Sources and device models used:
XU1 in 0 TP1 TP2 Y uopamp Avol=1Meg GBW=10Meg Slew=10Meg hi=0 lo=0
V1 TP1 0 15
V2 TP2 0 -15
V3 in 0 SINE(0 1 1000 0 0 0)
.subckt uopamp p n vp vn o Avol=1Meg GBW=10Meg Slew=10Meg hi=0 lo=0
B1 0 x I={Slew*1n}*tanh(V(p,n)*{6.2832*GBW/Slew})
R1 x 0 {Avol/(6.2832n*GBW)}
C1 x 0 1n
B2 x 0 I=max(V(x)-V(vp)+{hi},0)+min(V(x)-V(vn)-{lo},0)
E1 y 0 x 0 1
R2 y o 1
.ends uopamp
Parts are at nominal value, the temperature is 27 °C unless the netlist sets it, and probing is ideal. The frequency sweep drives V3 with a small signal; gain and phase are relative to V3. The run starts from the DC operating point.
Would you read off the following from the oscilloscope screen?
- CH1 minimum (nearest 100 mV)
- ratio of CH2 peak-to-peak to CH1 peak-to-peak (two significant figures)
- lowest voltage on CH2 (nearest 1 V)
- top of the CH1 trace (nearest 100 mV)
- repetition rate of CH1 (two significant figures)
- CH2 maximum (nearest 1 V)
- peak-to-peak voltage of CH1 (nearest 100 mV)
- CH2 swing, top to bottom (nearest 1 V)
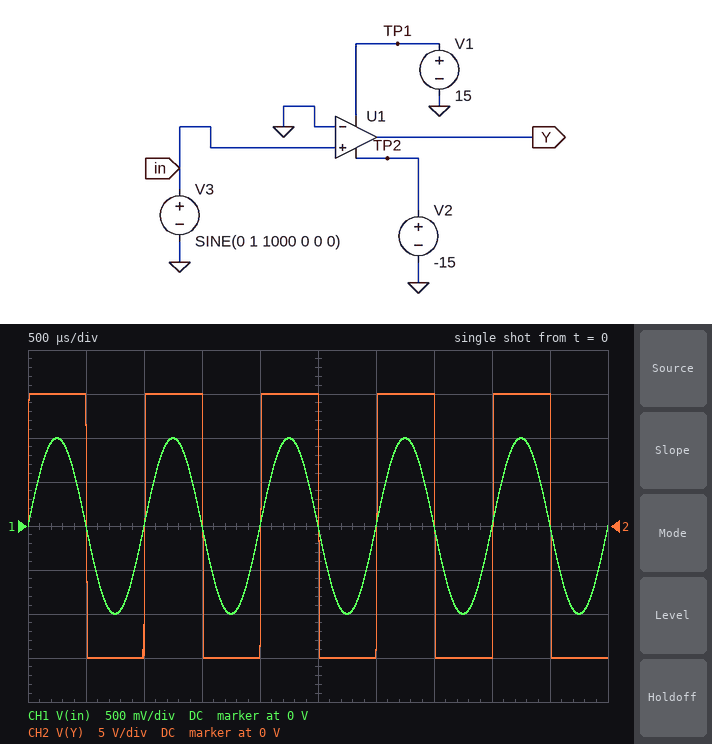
-1.0 V
15
-15 V
1.0 V
1.0 kHz
15 V
2.0 V
30 V
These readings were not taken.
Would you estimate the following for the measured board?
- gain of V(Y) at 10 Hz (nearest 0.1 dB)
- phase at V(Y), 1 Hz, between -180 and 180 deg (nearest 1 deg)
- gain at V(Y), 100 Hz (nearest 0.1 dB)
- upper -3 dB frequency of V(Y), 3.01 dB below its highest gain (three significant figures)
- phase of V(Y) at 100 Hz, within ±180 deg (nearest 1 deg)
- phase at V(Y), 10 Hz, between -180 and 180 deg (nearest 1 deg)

117.0 dB
-6 deg
100.0 dB
10.0 Hz
-84 deg
-45 deg
